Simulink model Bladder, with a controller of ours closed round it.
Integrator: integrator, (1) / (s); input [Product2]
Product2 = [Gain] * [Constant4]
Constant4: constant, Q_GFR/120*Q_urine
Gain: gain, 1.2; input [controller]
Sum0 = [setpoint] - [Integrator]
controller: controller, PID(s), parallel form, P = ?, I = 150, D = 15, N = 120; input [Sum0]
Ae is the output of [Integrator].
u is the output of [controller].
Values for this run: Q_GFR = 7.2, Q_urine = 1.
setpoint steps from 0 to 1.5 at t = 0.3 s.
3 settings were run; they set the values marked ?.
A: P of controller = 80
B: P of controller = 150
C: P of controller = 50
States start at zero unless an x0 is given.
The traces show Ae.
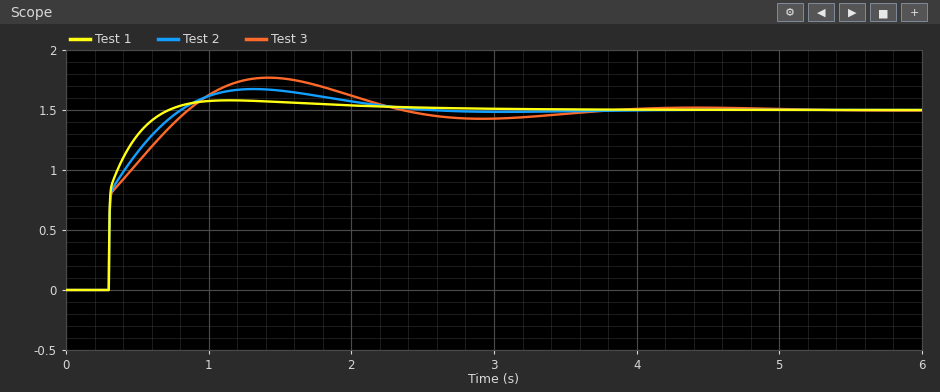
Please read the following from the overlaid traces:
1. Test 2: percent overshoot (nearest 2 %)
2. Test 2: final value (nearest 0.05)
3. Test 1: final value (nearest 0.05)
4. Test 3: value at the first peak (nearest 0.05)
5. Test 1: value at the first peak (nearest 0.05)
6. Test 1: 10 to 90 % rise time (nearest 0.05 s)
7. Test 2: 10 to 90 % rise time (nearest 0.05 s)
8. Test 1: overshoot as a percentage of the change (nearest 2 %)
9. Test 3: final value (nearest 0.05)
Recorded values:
12 %
1.50
1.50
1.75
1.60
0.25 s
0.35 s
6 %
1.50
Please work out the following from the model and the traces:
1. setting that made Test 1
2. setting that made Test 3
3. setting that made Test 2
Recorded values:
B
C
A
